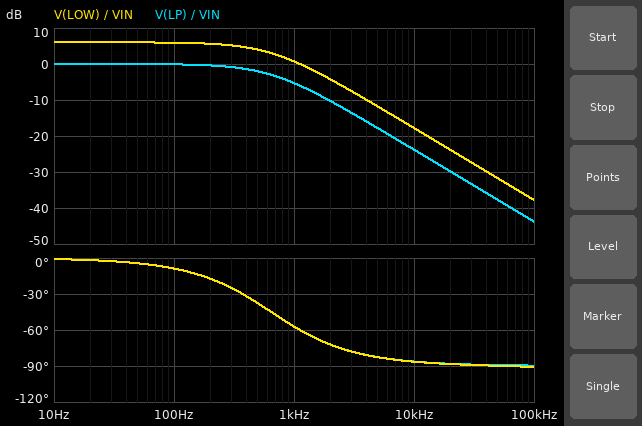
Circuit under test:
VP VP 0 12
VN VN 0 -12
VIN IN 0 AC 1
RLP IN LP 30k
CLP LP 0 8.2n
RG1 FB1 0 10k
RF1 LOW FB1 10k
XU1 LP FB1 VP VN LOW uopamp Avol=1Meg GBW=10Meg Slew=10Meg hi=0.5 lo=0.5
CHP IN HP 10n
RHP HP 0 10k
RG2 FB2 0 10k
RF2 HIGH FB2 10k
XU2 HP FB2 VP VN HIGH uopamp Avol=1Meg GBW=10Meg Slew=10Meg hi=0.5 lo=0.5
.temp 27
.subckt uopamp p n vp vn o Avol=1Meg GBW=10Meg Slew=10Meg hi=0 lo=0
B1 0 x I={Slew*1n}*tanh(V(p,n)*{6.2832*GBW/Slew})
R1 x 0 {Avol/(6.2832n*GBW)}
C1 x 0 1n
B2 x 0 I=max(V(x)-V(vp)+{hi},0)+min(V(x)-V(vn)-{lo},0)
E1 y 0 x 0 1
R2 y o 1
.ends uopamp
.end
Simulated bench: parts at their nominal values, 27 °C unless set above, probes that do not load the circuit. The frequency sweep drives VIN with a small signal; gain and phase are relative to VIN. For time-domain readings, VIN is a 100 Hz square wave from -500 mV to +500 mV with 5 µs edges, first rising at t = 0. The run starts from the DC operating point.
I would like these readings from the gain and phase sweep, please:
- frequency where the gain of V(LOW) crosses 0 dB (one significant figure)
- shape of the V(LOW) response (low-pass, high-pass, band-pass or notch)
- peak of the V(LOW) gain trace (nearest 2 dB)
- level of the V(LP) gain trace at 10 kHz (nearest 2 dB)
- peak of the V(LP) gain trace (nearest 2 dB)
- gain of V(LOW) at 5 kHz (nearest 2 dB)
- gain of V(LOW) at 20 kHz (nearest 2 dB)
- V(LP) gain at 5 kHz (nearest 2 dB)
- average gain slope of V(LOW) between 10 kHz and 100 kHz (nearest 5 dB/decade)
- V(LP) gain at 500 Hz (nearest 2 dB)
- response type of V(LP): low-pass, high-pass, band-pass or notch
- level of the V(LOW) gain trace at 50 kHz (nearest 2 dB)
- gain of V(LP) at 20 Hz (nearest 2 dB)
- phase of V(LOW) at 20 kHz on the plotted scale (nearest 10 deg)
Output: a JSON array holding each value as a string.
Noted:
["1 kHz", "low-pass", "6 dB", "-24 dB", "0 dB", "-12 dB", "-24 dB", "-18 dB", "-20 dB/decade", "-2 dB", "low-pass", "-32 dB", "0 dB", "-90 deg"]
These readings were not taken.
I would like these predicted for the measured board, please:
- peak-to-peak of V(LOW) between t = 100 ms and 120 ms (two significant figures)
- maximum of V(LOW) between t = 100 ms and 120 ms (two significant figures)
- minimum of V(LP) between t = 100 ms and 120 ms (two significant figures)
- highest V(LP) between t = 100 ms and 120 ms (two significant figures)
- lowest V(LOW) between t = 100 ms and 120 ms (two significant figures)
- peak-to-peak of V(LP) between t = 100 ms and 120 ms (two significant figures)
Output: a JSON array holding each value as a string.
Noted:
["2.0 V", "1.0 V", "-500 mV", "500 mV", "-1.0 V", "1.0 V"]
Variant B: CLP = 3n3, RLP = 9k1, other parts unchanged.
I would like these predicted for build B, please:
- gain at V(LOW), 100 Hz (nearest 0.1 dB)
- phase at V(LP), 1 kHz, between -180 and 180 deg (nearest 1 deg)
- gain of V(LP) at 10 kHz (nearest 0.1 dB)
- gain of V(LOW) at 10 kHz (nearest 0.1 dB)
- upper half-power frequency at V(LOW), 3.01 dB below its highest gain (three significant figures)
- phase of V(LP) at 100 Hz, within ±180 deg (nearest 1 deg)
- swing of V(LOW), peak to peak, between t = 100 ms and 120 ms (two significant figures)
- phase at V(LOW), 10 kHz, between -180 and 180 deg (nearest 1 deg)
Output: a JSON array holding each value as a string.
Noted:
["6.0 dB", "-11 deg", "-6.6 dB", "-0.6 dB", "5.30 kHz", "-1 deg", "2.0 V", "-62 deg"]
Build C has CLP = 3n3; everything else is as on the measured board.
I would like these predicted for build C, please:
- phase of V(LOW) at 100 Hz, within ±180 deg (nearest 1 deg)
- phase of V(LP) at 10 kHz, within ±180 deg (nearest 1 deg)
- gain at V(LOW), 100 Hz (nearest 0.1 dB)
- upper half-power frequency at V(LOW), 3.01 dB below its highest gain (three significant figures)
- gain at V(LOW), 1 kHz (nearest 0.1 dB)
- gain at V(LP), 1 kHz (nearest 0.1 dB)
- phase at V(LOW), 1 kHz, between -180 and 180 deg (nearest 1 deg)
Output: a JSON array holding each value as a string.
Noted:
["-4 deg", "-81 deg", "6.0 dB", "1.61 kHz", "4.6 dB", "-1.4 dB", "-32 deg"]
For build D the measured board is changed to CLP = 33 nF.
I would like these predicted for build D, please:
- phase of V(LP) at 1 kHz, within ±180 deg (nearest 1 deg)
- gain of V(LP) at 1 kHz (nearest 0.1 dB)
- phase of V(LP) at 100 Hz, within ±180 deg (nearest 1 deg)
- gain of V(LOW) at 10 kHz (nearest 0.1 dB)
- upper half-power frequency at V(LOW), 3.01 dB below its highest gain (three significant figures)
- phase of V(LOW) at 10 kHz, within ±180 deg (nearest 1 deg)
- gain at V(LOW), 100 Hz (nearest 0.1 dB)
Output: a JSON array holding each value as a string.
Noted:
["-81 deg", "-16.0 dB", "-32 deg", "-29.9 dB", "161 Hz", "-89 deg", "4.6 dB"]
